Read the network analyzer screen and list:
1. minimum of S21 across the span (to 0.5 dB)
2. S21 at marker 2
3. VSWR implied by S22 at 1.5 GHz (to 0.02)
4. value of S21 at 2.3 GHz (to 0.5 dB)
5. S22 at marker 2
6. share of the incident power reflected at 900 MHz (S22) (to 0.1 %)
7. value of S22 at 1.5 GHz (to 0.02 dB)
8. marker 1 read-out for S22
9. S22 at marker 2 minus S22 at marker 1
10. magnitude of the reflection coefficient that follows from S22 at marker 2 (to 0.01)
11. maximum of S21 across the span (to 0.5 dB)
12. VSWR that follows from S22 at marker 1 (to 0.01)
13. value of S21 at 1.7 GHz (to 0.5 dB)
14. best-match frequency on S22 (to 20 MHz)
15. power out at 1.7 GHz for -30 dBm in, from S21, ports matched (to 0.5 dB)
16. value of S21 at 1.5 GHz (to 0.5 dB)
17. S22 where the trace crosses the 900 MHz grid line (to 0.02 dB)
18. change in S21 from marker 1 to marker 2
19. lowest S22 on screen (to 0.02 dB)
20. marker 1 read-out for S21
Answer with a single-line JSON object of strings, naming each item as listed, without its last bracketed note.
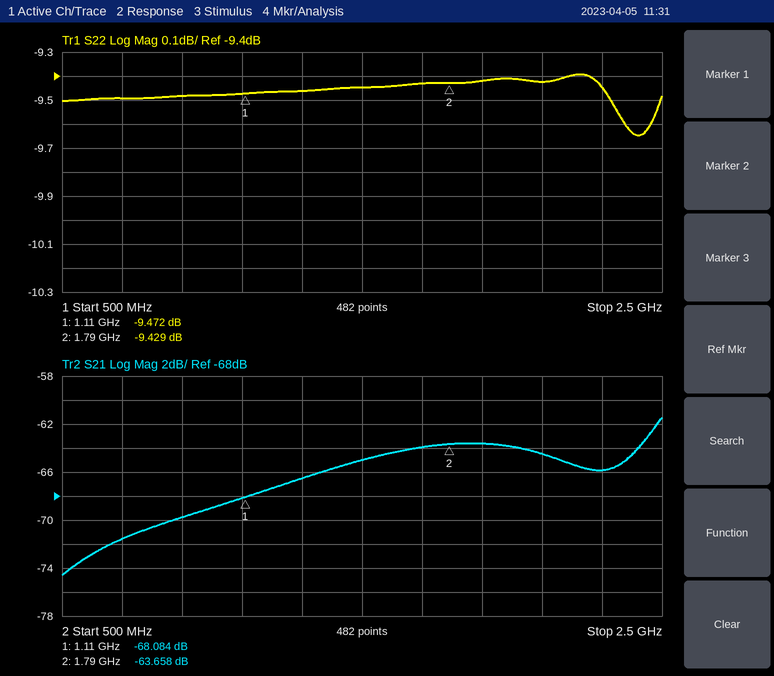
{"minimum of S21 across the span": "-74.5 dB", "S21 at marker 2": "-63.658 dB", "VSWR implied by S22 at 1.5 GHz": "2.02", "value of S21 at 2.3 GHz": "-66.0 dB", "S22 at marker 2": "-9.429 dB", "share of the incident power reflected at 900 MHz (S22)": "11.3 %", "value of S22 at 1.5 GHz": "-9.44 dB", "marker 1 read-out for S22": "-9.472 dB", "S22 at marker 2 minus S22 at marker 1": "0.043 dB", "magnitude of the reflection coefficient that follows from S22 at marker 2": "0.34", "maximum of S21 across the span": "-61.5 dB", "VSWR that follows from S22 at marker 1": "2.01", "value of S21 at 1.7 GHz": "-64.0 dB", "best-match frequency on S22": "2.42 GHz", "power out at 1.7 GHz for -30 dBm in, from S21, ports matched": "-94.0 dBm", "value of S21 at 1.5 GHz": "-65.0 dB", "S22 where the trace crosses the 900 MHz grid line": "-9.48 dB", "change in S21 from marker 1 to marker 2": "4.426 dB", "lowest S22 on screen": "-9.64 dB", "marker 1 read-out for S21": "-68.084 dB"}
